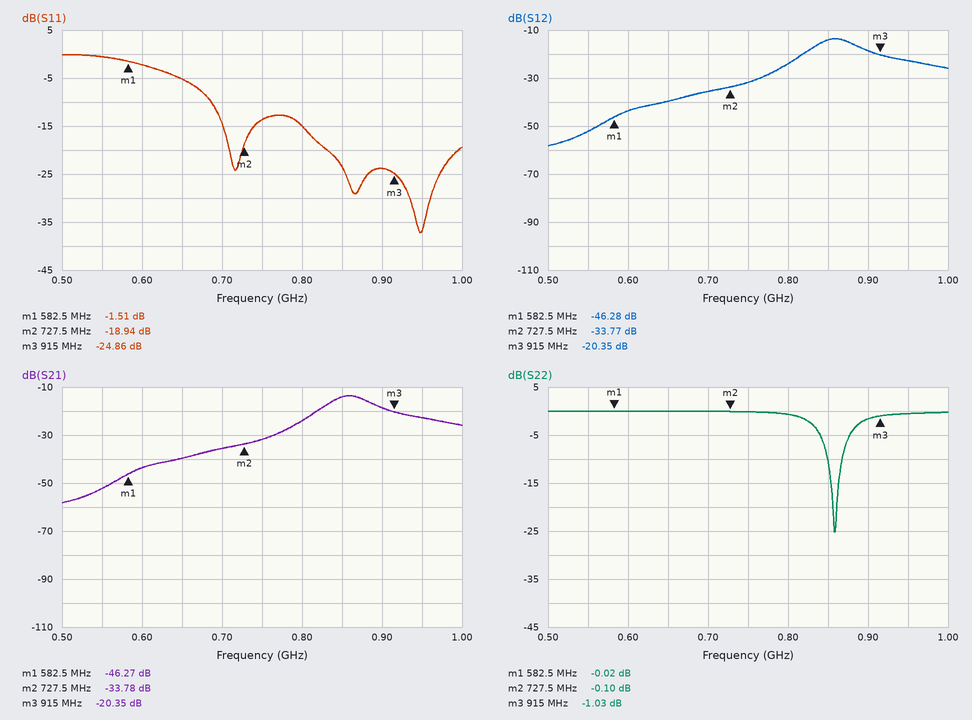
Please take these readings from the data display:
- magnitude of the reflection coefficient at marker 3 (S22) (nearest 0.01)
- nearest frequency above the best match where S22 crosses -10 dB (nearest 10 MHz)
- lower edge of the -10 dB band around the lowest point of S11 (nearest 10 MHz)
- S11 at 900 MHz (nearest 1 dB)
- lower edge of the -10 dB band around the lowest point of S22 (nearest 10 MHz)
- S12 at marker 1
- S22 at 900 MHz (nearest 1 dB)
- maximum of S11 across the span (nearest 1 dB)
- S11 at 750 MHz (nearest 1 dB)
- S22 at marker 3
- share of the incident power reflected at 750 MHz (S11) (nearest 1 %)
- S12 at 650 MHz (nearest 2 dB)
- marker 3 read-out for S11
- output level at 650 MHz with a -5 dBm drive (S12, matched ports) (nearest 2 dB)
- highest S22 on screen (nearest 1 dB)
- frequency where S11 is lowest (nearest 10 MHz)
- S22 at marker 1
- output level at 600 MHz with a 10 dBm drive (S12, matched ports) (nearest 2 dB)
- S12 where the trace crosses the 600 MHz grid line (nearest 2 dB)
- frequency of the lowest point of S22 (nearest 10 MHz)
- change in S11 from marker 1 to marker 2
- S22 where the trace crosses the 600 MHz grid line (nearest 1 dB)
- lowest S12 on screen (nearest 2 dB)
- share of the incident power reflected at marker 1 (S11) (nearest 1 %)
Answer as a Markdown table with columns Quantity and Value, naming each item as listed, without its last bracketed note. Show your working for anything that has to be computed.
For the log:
| Quantity | Value |
|---|---|
| magnitude of the reflection coefficient at marker 3 (S22) | 10^(-1.03/20) ≈ 0.89 |
| nearest frequency above the best match where S22 crosses -10 dB | 870 MHz |
| lower edge of the -10 dB band around the lowest point of S11 | 690 MHz |
| S11 at 900 MHz | -24 dB |
| lower edge of the -10 dB band around the lowest point of S22 | 850 MHz |
| S12 at marker 1 | -46.28 dB |
| S22 at 900 MHz | -2 dB |
| maximum of S11 across the span | 0 dB |
| S11 at 750 MHz | -14 dB |
| S22 at marker 3 | -1.03 dB |
| share of the incident power reflected at 750 MHz (S11) | 10^(-14/10) ≈ 4 % |
| S12 at 650 MHz | -40 dB |
| marker 3 read-out for S11 | -24.86 dB |
| output level at 650 MHz with a -5 dBm drive (S12, matched ports) | -5 dBm + (-40 dB) = -44 dBm |
| highest S22 on screen | 0 dB |
| frequency where S11 is lowest | 950 MHz |
| S22 at marker 1 | -0.02 dB |
| output level at 600 MHz with a 10 dBm drive (S12, matched ports) | 10 dBm + (-44 dB) = -34 dBm |
| S12 where the trace crosses the 600 MHz grid line | -44 dB |
| frequency of the lowest point of S22 | 860 MHz |
| change in S11 from marker 1 to marker 2 | -18.94 − (-1.51) = -17.43 dB |
| S22 where the trace crosses the 600 MHz grid line | 0 dB |
| lowest S12 on screen | -58 dB |
| share of the incident power reflected at marker 1 (S11) | 10^(-1.51/10) ≈ 71 % |
